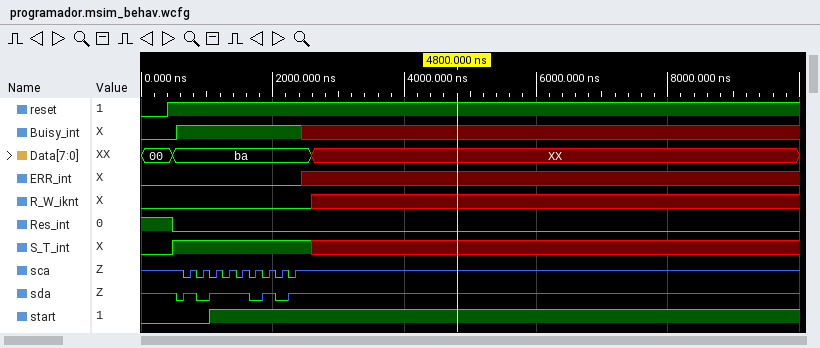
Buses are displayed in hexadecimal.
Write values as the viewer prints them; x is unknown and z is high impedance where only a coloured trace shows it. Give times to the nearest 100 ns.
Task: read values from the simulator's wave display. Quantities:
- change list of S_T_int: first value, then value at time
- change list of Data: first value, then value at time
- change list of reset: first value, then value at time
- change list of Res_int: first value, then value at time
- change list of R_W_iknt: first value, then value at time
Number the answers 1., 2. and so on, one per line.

1. 0, 1 at 500 ns, x at 2600 ns
2. 00, ba at 500 ns, XX at 2600 ns
3. 0, 1 at 400 ns
4. 1, 0 at 500 ns
5. 0, x at 2600 ns
